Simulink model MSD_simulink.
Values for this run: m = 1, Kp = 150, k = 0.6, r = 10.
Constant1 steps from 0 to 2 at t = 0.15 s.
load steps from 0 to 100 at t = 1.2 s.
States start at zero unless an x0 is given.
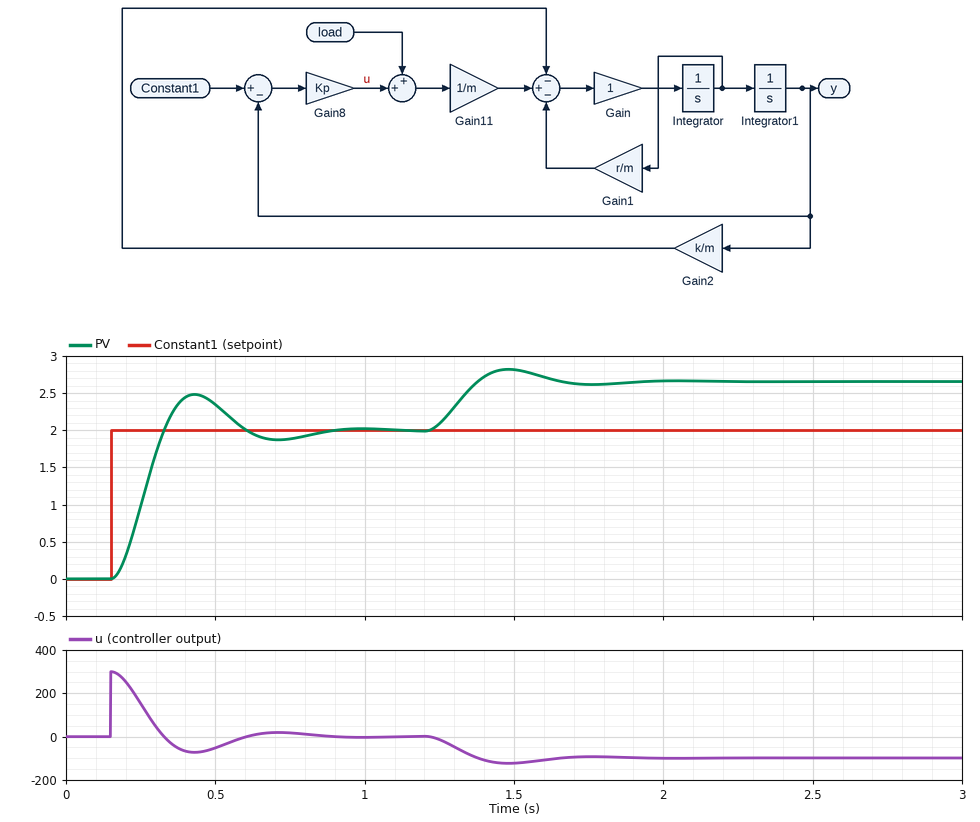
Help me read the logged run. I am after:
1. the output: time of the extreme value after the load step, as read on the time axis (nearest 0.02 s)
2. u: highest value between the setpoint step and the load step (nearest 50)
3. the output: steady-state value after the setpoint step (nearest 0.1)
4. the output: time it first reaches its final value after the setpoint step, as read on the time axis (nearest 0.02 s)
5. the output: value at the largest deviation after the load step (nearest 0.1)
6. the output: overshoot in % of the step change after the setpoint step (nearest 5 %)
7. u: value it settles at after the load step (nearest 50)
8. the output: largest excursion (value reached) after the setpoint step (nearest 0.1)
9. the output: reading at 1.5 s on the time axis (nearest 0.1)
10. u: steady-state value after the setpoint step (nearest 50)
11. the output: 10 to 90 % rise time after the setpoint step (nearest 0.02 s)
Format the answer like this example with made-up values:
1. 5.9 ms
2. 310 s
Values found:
1. 1.48 s
2. 300
3. 2.0
4. 0.32 s
5. 2.8
6. 25 %
7. -100
8. 2.5
9. 2.8
10. 0
11. 0.12 s
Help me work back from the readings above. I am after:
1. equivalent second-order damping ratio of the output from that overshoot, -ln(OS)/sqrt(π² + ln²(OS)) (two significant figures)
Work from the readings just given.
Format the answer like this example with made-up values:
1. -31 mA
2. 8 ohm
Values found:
1. 0.40
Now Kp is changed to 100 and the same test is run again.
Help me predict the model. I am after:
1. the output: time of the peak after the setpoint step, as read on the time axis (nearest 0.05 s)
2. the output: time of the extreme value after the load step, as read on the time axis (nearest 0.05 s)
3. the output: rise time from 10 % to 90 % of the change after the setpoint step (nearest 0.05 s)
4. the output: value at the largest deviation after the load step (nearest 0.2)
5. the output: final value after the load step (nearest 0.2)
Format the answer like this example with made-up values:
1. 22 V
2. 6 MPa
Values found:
1. 0.50 s
2. 1.55 s
3. 0.15 s
4. 3.2
5. 3.0
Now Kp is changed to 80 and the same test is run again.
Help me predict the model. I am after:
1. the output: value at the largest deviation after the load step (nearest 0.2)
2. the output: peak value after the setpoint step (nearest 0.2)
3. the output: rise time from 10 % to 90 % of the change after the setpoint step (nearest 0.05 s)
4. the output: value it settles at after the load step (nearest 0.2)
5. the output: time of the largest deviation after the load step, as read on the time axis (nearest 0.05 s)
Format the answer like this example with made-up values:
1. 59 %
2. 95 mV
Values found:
1. 3.4
2. 2.2
3. 0.20 s
4. 3.2
5. 1.60 s
